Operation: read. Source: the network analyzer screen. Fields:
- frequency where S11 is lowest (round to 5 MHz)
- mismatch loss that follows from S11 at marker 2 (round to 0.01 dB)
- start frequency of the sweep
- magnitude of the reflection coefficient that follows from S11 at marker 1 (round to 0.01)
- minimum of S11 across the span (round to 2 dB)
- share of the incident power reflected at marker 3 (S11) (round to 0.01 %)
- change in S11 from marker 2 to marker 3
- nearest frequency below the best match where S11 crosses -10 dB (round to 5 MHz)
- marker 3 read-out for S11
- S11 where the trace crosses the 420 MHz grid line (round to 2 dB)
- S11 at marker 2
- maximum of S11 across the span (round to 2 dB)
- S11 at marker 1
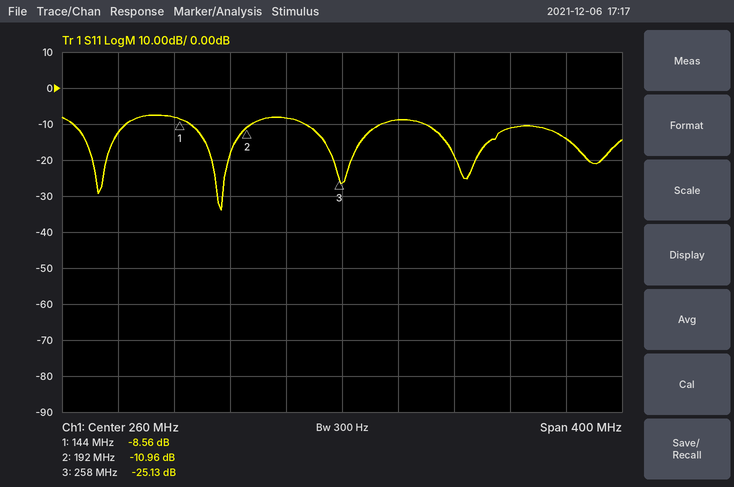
175 MHz
0.36 dB
60 MHz
0.37
-34 dB
0.31 %
-14.17 dB
150 MHz
-25.13 dB
-14 dB
-10.96 dB
-8 dB
-8.56 dB
